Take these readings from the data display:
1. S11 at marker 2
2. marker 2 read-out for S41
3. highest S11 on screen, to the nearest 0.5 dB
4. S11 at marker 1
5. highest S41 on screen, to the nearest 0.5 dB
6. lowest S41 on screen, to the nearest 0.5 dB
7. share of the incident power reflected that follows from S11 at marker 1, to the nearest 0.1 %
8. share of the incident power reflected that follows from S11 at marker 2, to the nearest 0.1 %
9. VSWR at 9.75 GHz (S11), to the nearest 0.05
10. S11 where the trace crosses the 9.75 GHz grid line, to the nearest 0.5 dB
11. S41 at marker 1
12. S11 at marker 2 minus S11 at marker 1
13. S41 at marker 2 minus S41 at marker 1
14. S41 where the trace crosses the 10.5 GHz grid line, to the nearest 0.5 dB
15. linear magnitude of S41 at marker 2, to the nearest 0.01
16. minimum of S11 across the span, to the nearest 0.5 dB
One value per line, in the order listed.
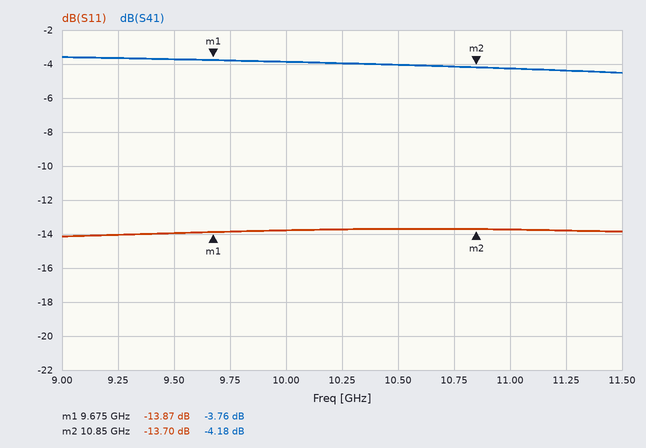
-13.70 dB
-4.18 dB
-13.5 dB
-13.87 dB
-3.5 dB
-4.5 dB
4.1 %
4.3 %
1.50
-14.0 dB
-3.76 dB
0.17 dB
-0.42 dB
-4.0 dB
0.62
-14.0 dB
